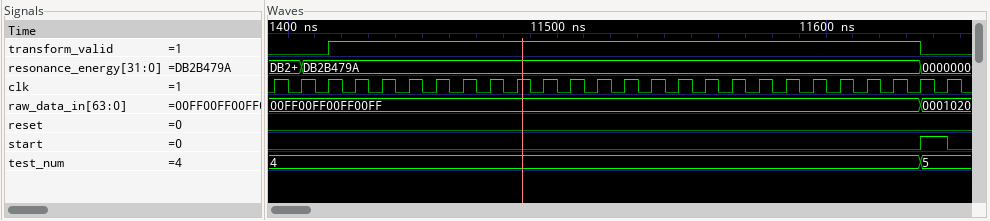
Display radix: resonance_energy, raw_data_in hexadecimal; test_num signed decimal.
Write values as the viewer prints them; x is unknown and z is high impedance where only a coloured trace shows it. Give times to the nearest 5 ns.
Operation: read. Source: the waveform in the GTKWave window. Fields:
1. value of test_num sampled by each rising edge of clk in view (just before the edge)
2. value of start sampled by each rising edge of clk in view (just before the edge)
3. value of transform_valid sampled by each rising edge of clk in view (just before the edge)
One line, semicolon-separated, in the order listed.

4, 4, 4, 4, 4, 4, 4, 4, 4, 4, 4, 4, 4, 4, 4, 4, 4, 4, 4, 4, 4, 4, 4, 4, 4, 5; 0 0 0 0 0 0 0 0 0 0 0 0 0 0 0 0 0 0 0 0 0 0 0 0 0 1; 0 0 0 1 1 1 1 1 1 1 1 1 1 1 1 1 1 1 1 1 1 1 1 1 1 0
